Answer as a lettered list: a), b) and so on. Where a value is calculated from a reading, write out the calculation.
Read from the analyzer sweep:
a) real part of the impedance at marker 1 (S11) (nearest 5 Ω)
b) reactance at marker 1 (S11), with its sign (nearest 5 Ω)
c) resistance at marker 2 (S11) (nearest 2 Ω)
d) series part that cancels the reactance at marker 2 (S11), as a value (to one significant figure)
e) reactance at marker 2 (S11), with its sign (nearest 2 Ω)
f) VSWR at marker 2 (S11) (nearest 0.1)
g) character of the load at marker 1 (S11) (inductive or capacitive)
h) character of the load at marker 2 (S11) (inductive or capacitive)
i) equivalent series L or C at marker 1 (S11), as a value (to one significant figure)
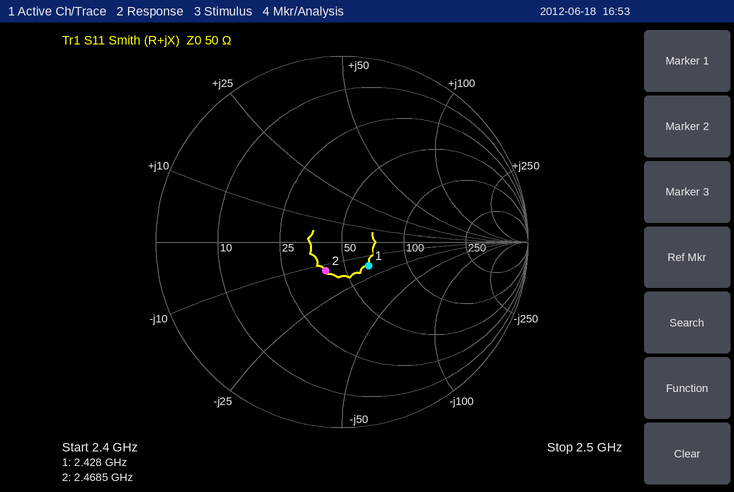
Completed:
a) 65 Ω
b) -15 Ω
c) 40 Ω
d) L = 12 Ω/(2π × 2.4685 GHz) ≈ 774 pH, so 800 pH to one significant figure
e) -12 Ω
f) 1.4
g) capacitive
h) capacitive
i) C = 1/(2π × 2.428 GHz × 15 Ω) ≈ 4 pF
